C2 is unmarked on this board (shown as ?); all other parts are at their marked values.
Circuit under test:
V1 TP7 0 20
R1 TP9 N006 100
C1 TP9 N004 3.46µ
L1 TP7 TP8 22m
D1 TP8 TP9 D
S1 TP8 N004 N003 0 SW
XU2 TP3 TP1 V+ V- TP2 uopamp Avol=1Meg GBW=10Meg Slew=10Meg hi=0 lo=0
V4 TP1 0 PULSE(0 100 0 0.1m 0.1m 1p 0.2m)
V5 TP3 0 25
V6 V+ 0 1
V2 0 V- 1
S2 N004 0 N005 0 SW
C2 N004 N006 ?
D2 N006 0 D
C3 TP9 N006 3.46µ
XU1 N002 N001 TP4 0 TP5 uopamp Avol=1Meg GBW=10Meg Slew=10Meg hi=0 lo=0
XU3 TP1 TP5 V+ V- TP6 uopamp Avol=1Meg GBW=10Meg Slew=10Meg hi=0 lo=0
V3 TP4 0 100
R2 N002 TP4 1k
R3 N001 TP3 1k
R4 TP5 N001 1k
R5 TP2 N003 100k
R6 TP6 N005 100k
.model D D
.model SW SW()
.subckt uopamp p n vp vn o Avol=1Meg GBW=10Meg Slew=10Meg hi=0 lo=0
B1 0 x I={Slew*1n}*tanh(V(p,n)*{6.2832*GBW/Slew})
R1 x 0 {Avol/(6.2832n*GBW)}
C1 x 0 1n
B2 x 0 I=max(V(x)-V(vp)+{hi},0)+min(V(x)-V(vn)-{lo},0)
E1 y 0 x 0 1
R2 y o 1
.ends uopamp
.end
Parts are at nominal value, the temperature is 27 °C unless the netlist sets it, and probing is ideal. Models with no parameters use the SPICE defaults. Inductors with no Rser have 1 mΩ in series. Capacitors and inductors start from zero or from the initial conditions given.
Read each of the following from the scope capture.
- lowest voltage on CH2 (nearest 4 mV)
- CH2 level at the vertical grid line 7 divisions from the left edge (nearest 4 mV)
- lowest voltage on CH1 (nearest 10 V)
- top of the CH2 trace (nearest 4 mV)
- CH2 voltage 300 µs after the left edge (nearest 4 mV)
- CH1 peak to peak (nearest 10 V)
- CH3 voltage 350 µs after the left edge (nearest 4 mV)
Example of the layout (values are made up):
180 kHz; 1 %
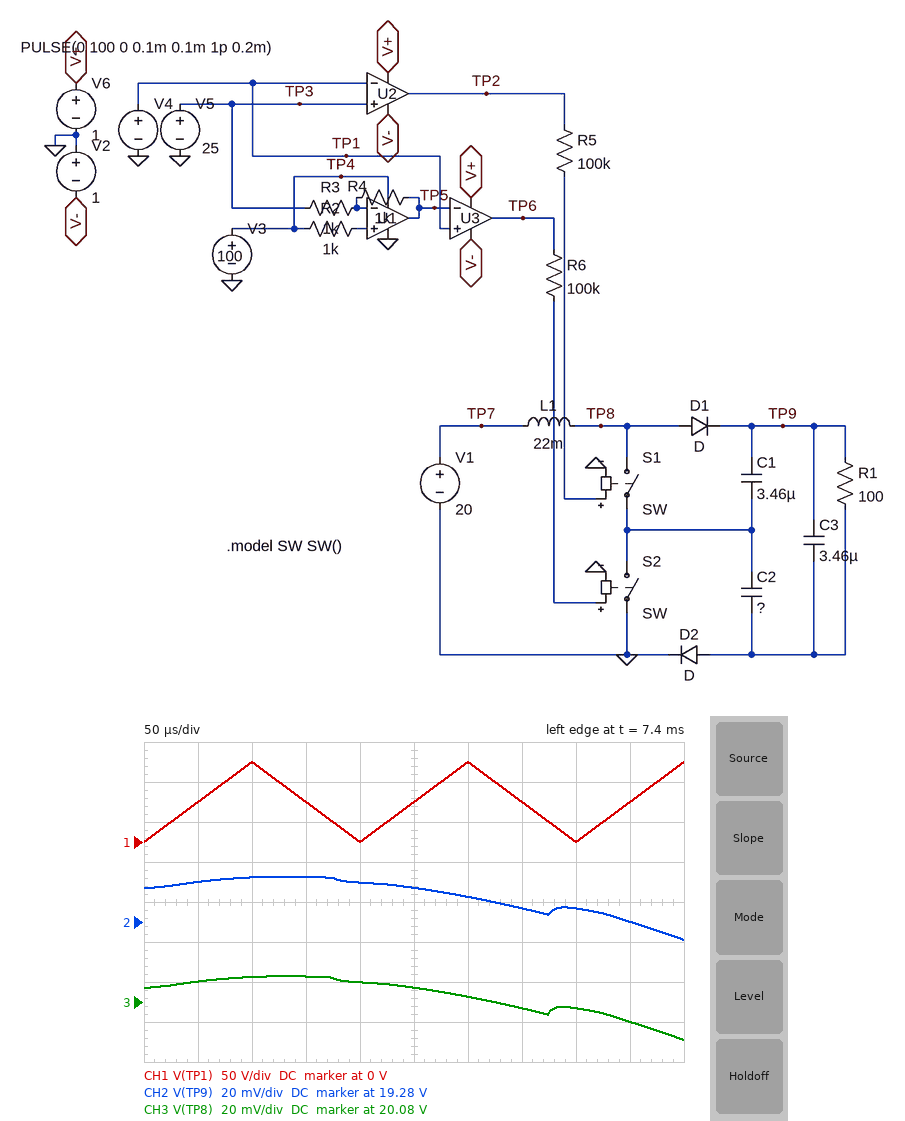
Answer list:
19.272 V; 19.288 V; 0 V; 19.304 V; 19.292 V; 100 V; 20.076 V
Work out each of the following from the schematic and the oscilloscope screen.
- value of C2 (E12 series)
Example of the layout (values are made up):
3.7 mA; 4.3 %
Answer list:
5.6 µF
